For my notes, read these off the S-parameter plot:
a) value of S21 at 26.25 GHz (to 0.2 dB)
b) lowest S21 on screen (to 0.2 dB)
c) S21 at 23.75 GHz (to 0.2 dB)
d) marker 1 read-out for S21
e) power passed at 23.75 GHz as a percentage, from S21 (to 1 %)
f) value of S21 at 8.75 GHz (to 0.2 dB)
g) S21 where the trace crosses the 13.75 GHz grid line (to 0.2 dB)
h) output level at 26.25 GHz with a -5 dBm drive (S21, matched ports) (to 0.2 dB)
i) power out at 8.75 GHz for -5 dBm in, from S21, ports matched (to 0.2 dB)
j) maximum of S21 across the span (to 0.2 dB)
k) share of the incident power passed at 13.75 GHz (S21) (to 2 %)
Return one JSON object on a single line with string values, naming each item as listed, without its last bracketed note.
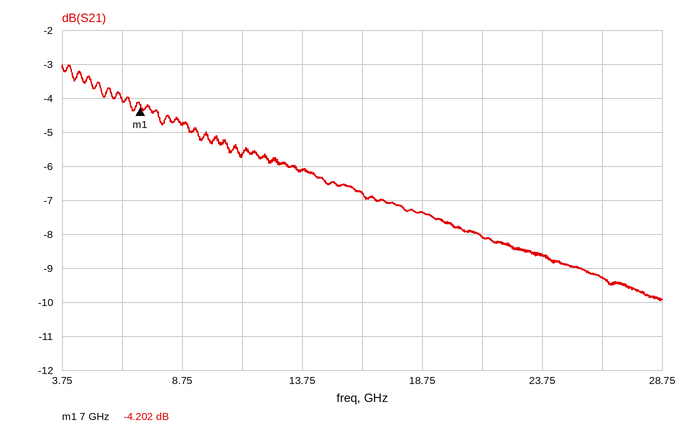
{"value of S21 at 26.25 GHz": "-9.2 dB", "lowest S21 on screen": "-10.0 dB", "S21 at 23.75 GHz": "-8.6 dB", "marker 1 read-out for S21": "-4.202 dB", "power passed at 23.75 GHz as a percentage, from S21": "14 %", "value of S21 at 8.75 GHz": "-4.8 dB", "S21 where the trace crosses the 13.75 GHz grid line": "-6.2 dB", "output level at 26.25 GHz with a -5 dBm drive (S21, matched ports)": "-14.2 dBm", "power out at 8.75 GHz for -5 dBm in, from S21, ports matched": "-9.8 dBm", "maximum of S21 across the span": "-3.0 dB", "share of the incident power passed at 13.75 GHz (S21)": "24 %"}
